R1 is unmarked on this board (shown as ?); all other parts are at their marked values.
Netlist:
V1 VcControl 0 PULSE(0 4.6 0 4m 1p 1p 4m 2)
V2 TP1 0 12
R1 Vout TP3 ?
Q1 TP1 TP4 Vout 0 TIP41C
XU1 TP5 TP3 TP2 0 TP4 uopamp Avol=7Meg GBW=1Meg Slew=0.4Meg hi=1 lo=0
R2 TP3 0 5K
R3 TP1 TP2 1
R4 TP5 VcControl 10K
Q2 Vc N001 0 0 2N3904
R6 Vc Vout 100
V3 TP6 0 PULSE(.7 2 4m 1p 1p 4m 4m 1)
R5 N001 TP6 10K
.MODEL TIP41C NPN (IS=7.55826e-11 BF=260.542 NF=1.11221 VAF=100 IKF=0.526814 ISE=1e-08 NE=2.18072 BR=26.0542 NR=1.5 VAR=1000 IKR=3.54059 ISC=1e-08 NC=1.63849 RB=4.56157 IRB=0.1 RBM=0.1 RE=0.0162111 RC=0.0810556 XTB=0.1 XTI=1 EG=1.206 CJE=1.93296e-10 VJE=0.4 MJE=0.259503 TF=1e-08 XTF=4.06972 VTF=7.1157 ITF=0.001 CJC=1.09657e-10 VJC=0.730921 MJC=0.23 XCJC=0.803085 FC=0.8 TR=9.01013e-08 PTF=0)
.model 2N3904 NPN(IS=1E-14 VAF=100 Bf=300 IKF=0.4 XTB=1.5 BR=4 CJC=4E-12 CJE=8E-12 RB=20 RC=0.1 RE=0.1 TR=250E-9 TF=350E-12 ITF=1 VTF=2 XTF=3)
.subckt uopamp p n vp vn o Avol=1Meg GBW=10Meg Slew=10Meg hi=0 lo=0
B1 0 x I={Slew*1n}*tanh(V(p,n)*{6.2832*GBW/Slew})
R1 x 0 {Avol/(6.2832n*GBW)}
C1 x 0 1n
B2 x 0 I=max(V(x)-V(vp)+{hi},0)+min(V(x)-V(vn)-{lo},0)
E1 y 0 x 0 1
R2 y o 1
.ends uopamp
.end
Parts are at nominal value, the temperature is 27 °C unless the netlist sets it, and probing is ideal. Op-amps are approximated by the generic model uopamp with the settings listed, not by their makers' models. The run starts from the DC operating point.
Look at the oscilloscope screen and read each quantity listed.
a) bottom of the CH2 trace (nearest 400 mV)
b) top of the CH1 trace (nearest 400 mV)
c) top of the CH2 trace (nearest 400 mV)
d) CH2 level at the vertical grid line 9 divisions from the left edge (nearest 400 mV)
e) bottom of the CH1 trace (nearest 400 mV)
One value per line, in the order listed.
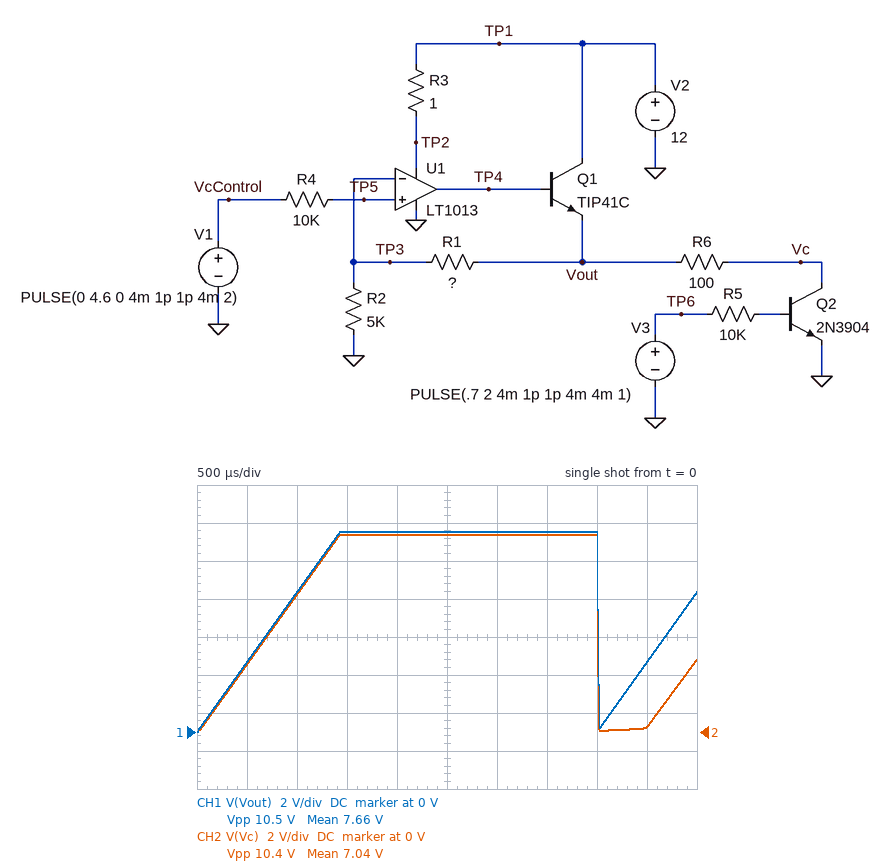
0 V
10.4 V
10.4 V
400 mV
0 V
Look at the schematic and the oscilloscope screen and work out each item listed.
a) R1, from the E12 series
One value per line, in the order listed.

27 kΩ
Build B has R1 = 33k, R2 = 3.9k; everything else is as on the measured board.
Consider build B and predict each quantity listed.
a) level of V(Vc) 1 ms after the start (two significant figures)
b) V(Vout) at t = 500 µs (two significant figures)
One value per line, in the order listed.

10 V
5.4 V
